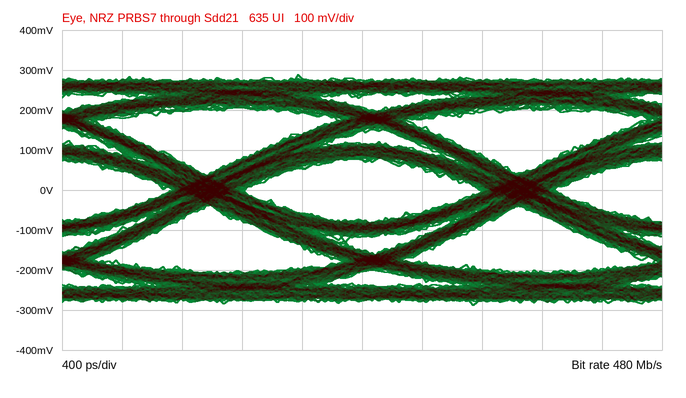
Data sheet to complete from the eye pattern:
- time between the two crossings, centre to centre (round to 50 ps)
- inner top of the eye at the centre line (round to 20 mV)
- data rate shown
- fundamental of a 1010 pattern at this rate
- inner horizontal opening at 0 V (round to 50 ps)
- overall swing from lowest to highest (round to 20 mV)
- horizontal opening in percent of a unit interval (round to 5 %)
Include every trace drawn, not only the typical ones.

2.10 ns
80 mV
480 Mb/s
240 MHz
1.55 ns
580 mV
75 %
